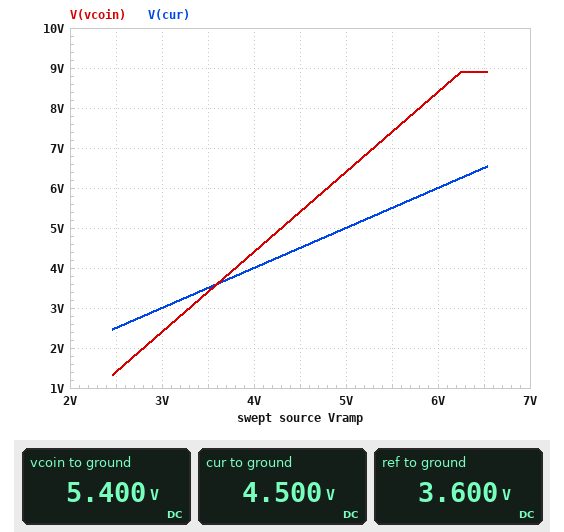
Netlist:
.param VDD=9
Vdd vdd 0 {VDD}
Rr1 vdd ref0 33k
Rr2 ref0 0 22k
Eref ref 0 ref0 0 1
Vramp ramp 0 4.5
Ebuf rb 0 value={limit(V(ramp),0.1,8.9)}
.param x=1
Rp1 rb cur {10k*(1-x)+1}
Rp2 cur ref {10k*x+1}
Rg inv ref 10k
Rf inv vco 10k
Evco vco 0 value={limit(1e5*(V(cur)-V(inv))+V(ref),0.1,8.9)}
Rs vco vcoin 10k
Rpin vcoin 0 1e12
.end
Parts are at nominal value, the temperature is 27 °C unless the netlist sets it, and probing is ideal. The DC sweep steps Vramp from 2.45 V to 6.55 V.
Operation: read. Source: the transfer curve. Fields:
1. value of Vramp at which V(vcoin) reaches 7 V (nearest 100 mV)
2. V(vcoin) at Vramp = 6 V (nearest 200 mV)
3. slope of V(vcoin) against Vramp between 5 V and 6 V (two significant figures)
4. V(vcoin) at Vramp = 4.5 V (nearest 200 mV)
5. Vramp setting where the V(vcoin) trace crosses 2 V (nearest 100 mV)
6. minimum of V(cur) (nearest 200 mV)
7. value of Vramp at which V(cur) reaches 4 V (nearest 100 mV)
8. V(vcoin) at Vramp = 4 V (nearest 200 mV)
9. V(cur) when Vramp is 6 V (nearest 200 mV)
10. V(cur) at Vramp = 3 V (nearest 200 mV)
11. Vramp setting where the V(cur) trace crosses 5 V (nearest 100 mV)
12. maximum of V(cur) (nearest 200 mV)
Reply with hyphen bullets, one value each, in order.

- 5.3 V
- 8.4 V
- 2.0 V/V
- 5.4 V
- 2.8 V
- 2.4 V
- 4.0 V
- 4.4 V
- 6.0 V
- 3.0 V
- 5.0 V
- 6.6 V
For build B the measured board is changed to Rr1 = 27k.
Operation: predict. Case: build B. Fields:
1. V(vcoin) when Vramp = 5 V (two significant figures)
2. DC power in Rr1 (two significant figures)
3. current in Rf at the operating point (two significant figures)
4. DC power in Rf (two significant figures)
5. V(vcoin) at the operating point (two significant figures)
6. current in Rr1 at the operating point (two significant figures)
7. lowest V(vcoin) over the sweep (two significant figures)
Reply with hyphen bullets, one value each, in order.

- 6.0 V
- 910 µW
- 46 µA
- 21 µW
- 5.0 V
- 180 µA
- 870 mV
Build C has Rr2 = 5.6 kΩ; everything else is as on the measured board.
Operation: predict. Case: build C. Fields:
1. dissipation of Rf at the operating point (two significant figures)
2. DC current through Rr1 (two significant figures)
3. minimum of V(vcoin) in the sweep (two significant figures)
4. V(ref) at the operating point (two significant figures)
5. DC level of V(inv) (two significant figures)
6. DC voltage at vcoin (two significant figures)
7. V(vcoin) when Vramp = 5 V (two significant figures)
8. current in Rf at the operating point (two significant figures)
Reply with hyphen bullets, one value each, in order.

- 1.0 mW
- 230 µA
- 3.6 V
- 1.3 V
- 4.5 V
- 7.7 V
- 8.7 V
- 320 µA
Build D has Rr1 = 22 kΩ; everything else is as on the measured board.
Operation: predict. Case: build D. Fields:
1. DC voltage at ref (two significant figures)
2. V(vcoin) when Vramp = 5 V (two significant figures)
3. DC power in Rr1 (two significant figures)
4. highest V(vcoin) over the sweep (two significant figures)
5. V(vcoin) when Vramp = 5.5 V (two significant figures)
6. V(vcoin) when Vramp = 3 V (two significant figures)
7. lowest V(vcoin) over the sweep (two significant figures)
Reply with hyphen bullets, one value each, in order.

- 4.5 V
- 5.5 V
- 920 µW
- 8.6 V
- 6.5 V
- 1.5 V
- 410 mV
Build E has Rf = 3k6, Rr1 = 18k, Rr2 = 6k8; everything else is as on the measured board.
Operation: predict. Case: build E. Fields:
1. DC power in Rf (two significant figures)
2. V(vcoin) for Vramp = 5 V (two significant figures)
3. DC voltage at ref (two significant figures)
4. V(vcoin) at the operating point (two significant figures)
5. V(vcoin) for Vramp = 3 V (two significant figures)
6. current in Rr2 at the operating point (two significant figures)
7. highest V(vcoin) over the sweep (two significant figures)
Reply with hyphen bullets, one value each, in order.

- 150 µW
- 5.9 V
- 2.5 V
- 5.2 V
- 3.2 V
- 360 µA
- 8.0 V
